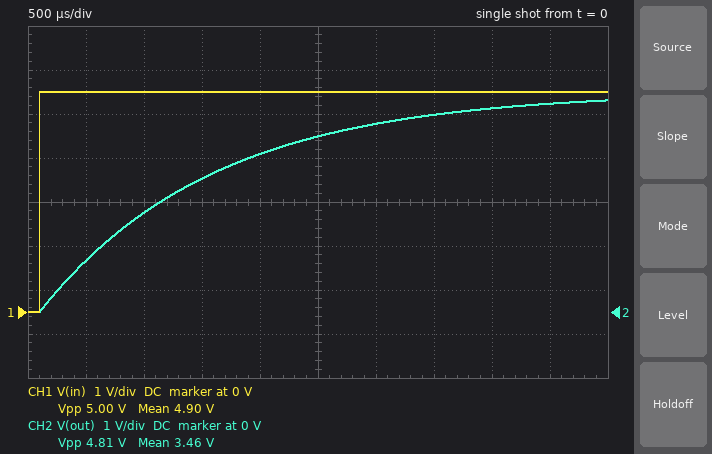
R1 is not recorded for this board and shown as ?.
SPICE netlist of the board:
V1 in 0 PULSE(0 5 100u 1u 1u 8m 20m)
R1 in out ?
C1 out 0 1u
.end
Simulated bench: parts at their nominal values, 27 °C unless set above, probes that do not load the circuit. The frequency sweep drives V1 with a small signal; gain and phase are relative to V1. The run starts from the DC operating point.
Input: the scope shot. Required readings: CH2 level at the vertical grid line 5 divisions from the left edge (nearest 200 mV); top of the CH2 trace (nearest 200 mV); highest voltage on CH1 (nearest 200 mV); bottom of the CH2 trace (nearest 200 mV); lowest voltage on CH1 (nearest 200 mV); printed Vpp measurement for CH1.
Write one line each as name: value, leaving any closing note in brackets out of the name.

CH2 level at the vertical grid line 5 divisions from the left edge: 4.0 V
top of the CH2 trace: 4.8 V
highest voltage on CH1: 5.0 V
bottom of the CH2 trace: 0 V
lowest voltage on CH1: 0 V
printed Vpp measurement for CH1: 5.00 V
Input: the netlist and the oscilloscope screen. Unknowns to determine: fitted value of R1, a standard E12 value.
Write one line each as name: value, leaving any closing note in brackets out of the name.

fitted value of R1, a standard E12 value: 1.5 kΩ
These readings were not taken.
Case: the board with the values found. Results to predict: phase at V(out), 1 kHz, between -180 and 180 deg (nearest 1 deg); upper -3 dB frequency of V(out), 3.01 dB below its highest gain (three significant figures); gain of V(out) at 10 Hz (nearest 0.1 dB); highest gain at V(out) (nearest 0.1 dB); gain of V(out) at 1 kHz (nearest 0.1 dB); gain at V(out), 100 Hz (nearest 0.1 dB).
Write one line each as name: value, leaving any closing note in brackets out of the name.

phase at V(out), 1 kHz, between -180 and 180 deg: -84 deg
upper -3 dB frequency of V(out), 3.01 dB below its highest gain: 106 Hz
gain of V(out) at 10 Hz: 0 dB
highest gain at V(out): 0 dB
gain of V(out) at 1 kHz: -19.5 dB
gain at V(out), 100 Hz: -2.8 dB
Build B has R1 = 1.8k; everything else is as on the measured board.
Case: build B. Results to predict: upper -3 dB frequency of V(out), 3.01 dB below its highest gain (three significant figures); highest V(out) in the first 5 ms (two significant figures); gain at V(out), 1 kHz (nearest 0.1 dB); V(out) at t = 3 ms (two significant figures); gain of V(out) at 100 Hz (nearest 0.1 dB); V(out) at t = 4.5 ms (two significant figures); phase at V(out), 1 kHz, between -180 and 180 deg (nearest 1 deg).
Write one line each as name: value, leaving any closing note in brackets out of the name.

upper -3 dB frequency of V(out), 3.01 dB below its highest gain: 88.4 Hz
highest V(out) in the first 5 ms: 4.7 V
gain at V(out), 1 kHz: -21.1 dB
V(out) at t = 3 ms: 4.0 V
gain of V(out) at 100 Hz: -3.6 dB
V(out) at t = 4.5 ms: 4.6 V
phase at V(out), 1 kHz, between -180 and 180 deg: -85 deg
